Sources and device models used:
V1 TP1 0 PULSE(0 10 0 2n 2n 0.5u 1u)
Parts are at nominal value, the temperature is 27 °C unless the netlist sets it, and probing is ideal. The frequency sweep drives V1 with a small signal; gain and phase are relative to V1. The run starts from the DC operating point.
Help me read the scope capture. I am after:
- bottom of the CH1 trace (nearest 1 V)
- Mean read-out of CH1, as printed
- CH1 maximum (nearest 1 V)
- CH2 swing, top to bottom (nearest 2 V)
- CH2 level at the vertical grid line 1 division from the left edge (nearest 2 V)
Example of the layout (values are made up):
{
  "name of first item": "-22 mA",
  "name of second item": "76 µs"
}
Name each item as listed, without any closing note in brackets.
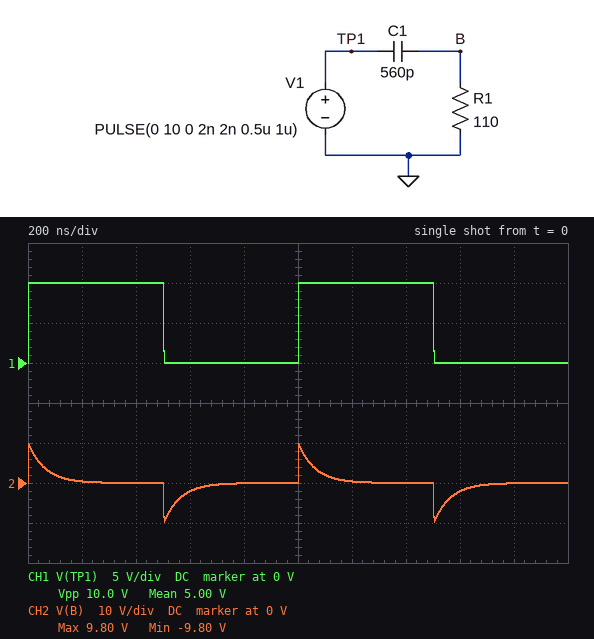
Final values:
{
  "bottom of the CH1 trace": "0 V",
  "Mean read-out of CH1, as printed": "5.00 V",
  "CH1 maximum": "10 V",
  "CH2 swing, top to bottom": "20 V",
  "CH2 level at the vertical grid line 1 division from the left edge": "0 V"
}
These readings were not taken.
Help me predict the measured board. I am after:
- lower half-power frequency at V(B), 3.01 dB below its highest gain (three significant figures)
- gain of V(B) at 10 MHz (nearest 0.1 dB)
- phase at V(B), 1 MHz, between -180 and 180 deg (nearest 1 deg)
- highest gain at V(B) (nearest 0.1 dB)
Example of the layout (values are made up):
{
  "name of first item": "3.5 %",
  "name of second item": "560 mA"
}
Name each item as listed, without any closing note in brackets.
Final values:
{
  "lower half-power frequency at V(B), 3.01 dB below its highest gain": "2.58 MHz",
  "gain of V(B) at 10 MHz": "-0.3 dB",
  "phase at V(B), 1 MHz, between -180 and 180 deg": "69 deg",
  "highest gain at V(B)": "0 dB"
}
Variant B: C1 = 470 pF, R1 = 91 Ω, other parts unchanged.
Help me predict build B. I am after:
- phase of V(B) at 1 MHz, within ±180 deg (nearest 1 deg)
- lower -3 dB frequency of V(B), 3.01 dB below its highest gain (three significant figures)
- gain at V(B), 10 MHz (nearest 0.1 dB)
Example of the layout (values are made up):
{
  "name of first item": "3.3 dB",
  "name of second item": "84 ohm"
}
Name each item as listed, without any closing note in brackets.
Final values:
{
  "phase of V(B) at 1 MHz, within ±180 deg": "75 deg",
  "lower -3 dB frequency of V(B), 3.01 dB below its highest gain": "3.72 MHz",
  "gain at V(B), 10 MHz": "-0.6 dB"
}
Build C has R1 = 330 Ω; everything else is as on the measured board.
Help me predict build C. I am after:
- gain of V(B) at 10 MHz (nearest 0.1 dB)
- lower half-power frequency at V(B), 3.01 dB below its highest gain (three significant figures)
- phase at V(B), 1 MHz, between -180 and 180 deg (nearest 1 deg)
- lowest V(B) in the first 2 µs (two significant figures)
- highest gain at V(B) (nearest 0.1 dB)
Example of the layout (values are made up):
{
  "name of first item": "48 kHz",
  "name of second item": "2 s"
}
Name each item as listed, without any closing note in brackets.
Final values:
{
  "gain of V(B) at 10 MHz": "0 dB",
  "lower half-power frequency at V(B), 3.01 dB below its highest gain": "861 kHz",
  "phase at V(B), 1 MHz, between -180 and 180 deg": "41 deg",
  "lowest V(B) in the first 2 µs": "-9.3 V",
  "highest gain at V(B)": "0 dB"
}
